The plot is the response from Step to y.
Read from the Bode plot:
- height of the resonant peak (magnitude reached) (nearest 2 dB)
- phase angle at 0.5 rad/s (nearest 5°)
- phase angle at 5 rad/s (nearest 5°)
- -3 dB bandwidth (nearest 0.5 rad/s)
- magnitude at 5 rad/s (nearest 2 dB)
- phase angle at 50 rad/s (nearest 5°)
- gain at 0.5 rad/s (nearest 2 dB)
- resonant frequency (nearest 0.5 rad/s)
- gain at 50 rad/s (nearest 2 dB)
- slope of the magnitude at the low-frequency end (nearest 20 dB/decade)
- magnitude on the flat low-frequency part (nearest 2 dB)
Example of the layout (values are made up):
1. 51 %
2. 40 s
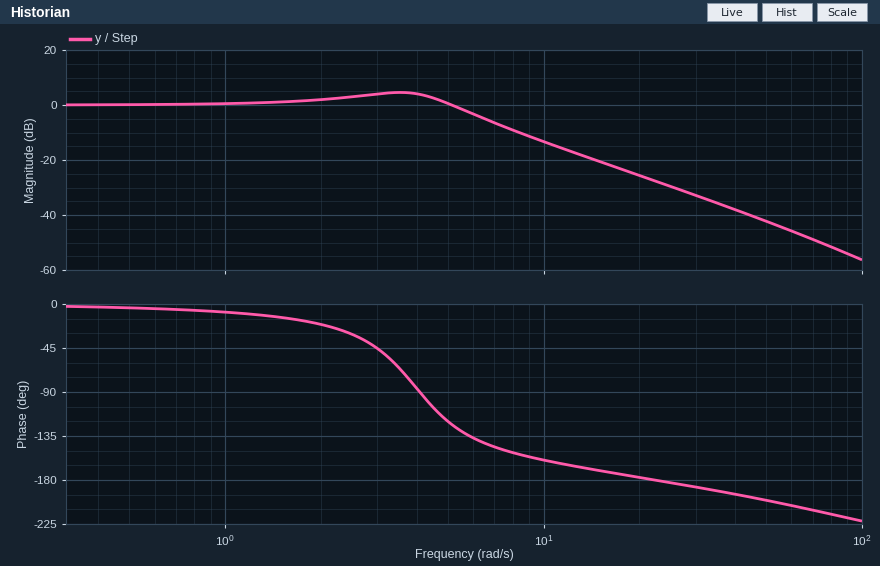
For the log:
1. 4 dB
2. -5°
3. -120°
4. 6.0 rad/s
5. 0 dB
6. -200°
7. 0 dB
8. 3.5 rad/s
9. -42 dB
10. 0 dB/decade
11. 0 dB
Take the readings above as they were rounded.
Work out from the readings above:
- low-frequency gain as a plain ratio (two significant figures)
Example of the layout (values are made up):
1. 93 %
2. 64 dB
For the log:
1. 1.0
